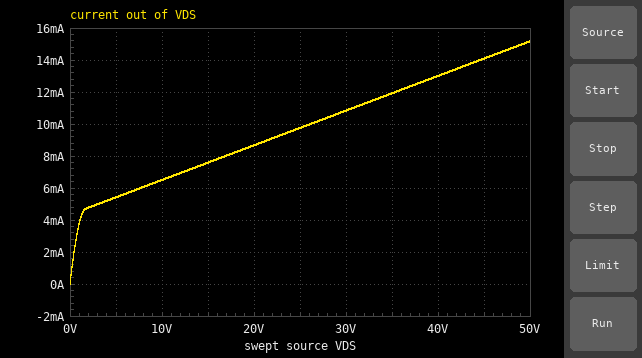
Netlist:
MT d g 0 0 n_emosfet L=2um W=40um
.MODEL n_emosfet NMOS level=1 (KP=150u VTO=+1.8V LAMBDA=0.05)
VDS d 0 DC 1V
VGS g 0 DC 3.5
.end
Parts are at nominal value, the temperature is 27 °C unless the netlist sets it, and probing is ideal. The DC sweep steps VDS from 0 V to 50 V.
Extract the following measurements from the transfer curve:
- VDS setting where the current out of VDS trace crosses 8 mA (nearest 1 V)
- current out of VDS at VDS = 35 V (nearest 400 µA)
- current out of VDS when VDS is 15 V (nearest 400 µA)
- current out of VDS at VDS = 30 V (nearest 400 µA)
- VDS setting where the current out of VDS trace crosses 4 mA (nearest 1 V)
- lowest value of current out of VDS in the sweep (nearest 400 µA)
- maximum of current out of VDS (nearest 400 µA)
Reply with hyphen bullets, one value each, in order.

- 17 V
- 12.0 mA
- 7.6 mA
- 10.8 mA
- 1 V
- 0 A
- 15.2 mA
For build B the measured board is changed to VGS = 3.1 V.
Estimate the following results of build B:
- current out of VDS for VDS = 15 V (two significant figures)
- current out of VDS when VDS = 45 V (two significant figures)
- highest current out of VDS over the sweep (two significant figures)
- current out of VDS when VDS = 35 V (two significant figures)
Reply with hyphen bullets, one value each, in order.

- 4.4 mA
- 8.2 mA
- 8.9 mA
- 7.0 mA
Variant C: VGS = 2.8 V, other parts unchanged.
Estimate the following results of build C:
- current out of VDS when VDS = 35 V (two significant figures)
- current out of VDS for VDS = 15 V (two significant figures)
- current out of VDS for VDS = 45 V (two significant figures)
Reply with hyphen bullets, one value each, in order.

- 4.1 mA
- 2.6 mA
- 4.9 mA
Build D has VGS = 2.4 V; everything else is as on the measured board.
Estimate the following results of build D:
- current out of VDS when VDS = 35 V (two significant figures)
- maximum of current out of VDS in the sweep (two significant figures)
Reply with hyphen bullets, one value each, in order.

- 1.5 mA
- 1.9 mA
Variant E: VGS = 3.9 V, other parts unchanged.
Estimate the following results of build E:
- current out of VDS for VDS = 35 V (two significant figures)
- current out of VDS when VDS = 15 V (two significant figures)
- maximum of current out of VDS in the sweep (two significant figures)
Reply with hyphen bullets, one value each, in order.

- 18 mA
- 12 mA
- 23 mA
